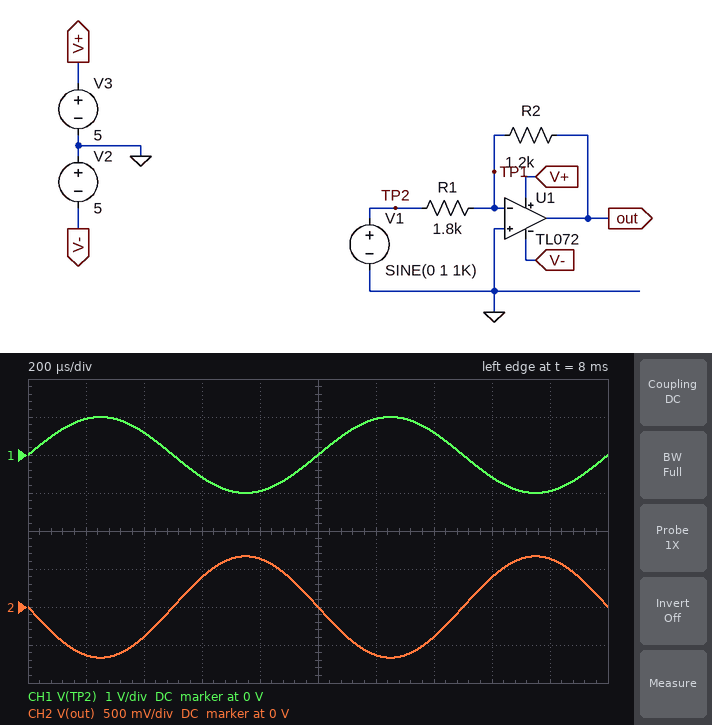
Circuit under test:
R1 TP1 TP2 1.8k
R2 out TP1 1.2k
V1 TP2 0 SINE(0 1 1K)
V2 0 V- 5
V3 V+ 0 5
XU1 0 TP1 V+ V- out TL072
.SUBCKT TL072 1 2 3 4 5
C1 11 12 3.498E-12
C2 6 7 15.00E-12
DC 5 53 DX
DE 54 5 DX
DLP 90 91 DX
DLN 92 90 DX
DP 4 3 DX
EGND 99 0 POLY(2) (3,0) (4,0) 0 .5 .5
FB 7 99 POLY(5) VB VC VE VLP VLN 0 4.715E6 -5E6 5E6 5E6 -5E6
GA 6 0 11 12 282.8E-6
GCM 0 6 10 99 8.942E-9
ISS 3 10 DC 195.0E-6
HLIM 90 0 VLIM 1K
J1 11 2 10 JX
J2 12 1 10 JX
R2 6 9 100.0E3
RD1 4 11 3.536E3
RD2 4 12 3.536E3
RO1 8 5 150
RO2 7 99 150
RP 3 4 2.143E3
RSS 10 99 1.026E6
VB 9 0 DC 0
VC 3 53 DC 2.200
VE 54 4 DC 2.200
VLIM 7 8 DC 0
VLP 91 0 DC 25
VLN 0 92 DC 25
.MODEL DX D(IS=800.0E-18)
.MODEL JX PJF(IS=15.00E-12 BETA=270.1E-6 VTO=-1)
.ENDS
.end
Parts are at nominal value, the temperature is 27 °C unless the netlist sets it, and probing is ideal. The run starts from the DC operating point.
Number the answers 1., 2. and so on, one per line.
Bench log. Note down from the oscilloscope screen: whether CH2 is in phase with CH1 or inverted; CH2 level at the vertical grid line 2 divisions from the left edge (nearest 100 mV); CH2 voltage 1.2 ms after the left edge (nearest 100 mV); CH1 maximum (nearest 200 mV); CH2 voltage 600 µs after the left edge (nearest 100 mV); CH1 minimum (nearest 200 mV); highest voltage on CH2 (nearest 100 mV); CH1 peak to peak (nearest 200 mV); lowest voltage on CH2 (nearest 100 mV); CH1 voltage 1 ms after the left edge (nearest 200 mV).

1. inverted
2. -400 mV
3. -600 mV
4. 1.0 V
5. 400 mV
6. -1.0 V
7. 700 mV
8. 2.0 V
9. -700 mV
10. 0 V
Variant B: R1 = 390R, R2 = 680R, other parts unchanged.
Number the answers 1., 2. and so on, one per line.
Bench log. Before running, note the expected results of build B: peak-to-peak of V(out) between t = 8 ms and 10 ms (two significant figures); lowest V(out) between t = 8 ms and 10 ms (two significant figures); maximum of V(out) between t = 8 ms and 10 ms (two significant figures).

1. 3.5 V
2. -1.7 V
3. 1.7 V
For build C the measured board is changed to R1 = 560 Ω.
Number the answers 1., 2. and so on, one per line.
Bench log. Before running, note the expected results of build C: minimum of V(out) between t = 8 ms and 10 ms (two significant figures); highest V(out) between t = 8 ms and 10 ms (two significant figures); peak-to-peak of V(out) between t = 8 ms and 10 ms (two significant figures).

1. -2.1 V
2. 2.1 V
3. 4.3 V
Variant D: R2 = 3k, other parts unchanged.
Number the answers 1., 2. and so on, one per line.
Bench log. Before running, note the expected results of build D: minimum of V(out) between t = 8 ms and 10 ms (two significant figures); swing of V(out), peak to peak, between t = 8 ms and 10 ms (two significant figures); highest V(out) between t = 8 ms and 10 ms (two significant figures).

1. -1.7 V
2. 3.3 V
3. 1.7 V
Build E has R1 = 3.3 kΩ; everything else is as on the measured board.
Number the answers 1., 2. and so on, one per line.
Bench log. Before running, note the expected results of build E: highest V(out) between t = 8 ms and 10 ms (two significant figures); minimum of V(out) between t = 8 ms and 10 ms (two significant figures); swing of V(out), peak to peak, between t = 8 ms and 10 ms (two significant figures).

1. 360 mV
2. -360 mV
3. 730 mV
